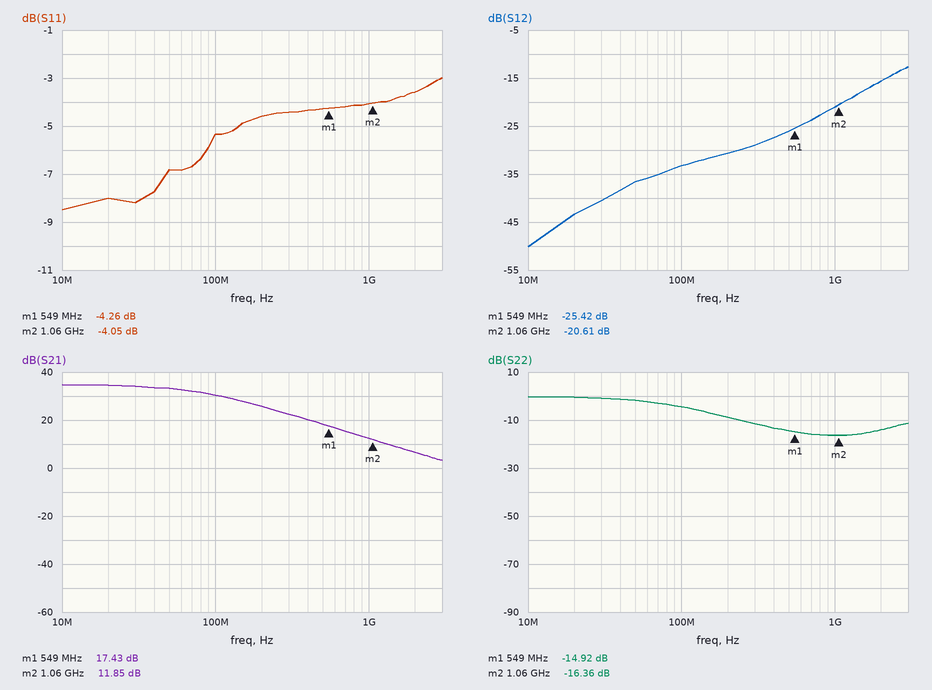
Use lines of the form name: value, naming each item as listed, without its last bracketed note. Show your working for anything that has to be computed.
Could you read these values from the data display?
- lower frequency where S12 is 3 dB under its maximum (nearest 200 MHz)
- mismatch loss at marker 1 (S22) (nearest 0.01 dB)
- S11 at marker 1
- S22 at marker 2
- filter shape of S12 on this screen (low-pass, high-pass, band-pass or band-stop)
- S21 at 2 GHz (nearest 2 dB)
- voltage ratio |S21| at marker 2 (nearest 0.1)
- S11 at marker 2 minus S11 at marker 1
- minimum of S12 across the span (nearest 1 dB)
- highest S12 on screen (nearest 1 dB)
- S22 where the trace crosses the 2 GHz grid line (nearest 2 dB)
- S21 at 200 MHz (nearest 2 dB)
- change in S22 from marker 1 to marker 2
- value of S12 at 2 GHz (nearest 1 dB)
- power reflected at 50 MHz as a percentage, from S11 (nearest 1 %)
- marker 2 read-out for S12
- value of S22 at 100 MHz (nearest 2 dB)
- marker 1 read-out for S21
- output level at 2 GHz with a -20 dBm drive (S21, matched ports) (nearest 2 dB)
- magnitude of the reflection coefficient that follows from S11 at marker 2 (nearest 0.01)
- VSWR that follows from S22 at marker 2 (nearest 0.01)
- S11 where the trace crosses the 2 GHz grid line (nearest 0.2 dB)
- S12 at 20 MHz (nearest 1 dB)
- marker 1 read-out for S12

lower frequency where S12 is 3 dB under its maximum: 2.0 GHz
mismatch loss at marker 1 (S22): −10 log10(1 − 10^(-14.92/10)) ≈ 0.14 dB
S11 at marker 1: -4.26 dB
S22 at marker 2: -16.36 dB
filter shape of S12 on this screen: high-pass
S21 at 2 GHz: 6 dB
voltage ratio |S21| at marker 2: 10^(11.85/20) ≈ 3.9
S11 at marker 2 minus S11 at marker 1: -4.05 − (-4.26) = 0.21 dB
minimum of S12 across the span: -50 dB
highest S12 on screen: -13 dB
S22 where the trace crosses the 2 GHz grid line: -14 dB
S21 at 200 MHz: 26 dB
change in S22 from marker 1 to marker 2: -16.36 − (-14.92) = -1.44 dB
value of S12 at 2 GHz: -16 dB
power reflected at 50 MHz as a percentage, from S11: 10^(-6.8/10) ≈ 21 %
marker 2 read-out for S12: -20.61 dB
value of S22 at 100 MHz: -4 dB
marker 1 read-out for S21: 17.43 dB
output level at 2 GHz with a -20 dBm drive (S21, matched ports): -20 dBm + (6 dB) = -14 dBm
magnitude of the reflection coefficient that follows from S11 at marker 2: 10^(-4.05/20) ≈ 0.63
VSWR that follows from S22 at marker 2: (1 + 0.1521)/(1 − 0.1521) ≈ 1.36
S11 where the trace crosses the 2 GHz grid line: -3.6 dB
S12 at 20 MHz: -43 dB
marker 1 read-out for S12: -25.42 dB
